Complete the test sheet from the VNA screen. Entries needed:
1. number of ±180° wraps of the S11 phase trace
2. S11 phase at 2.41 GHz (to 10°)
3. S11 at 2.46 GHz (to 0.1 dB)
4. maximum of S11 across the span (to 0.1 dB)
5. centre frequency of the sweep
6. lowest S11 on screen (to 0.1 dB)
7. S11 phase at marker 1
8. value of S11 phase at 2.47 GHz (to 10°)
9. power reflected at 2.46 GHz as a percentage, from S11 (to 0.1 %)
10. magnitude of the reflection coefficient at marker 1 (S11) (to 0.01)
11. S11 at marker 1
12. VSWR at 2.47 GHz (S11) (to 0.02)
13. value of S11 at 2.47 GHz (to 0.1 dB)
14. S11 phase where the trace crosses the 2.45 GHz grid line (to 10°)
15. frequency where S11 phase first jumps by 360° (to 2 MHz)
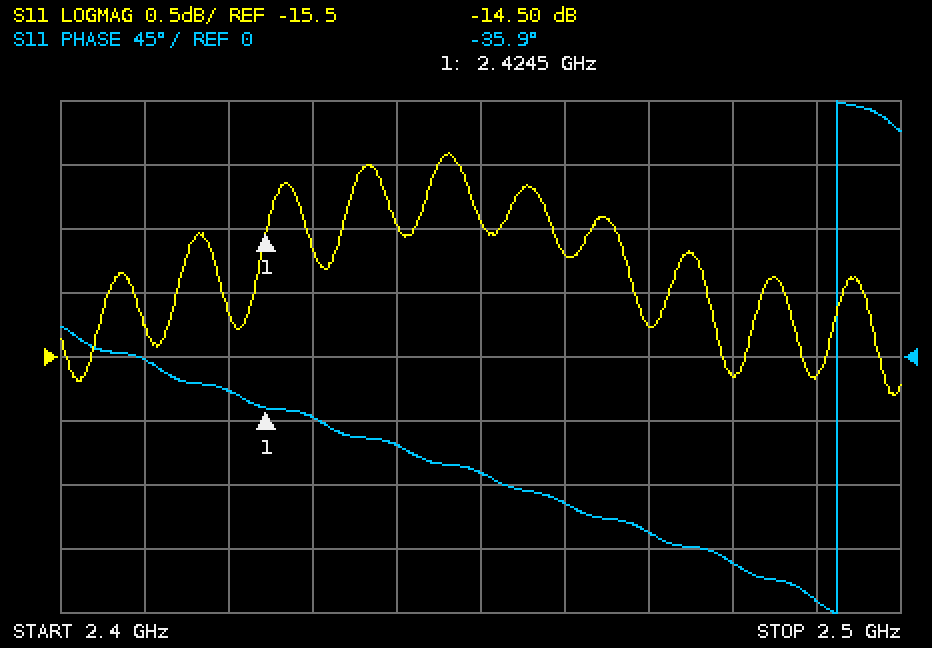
1
0°
-14.7 dB
-13.9 dB
2.45 GHz
-15.8 dB
-35.9°
-120°
3.4 %
0.19
-14.50 dB
1.42
-15.3 dB
-80°
2.492 GHz
